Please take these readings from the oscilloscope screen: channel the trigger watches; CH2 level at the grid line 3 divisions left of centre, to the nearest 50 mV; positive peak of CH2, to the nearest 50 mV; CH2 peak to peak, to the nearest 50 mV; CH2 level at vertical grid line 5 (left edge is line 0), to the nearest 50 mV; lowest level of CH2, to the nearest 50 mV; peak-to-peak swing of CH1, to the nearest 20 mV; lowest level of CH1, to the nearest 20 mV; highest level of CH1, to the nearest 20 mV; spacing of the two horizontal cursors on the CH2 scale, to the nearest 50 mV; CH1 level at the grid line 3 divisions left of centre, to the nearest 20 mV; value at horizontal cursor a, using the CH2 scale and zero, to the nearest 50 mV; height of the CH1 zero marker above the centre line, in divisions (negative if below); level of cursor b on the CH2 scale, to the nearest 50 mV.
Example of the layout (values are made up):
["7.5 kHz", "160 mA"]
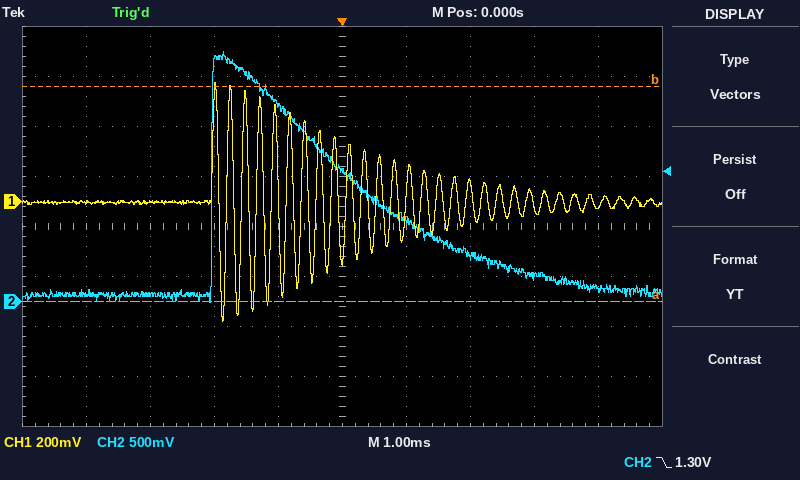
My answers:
["CH2", "50 mV", "2.50 V", "2.50 V", "1.30 V", "0 mV", "960 mV", "-480 mV", "480 mV", "2.15 V", "0 mV", "0 mV", "+0.5 div", "2.15 V"]
